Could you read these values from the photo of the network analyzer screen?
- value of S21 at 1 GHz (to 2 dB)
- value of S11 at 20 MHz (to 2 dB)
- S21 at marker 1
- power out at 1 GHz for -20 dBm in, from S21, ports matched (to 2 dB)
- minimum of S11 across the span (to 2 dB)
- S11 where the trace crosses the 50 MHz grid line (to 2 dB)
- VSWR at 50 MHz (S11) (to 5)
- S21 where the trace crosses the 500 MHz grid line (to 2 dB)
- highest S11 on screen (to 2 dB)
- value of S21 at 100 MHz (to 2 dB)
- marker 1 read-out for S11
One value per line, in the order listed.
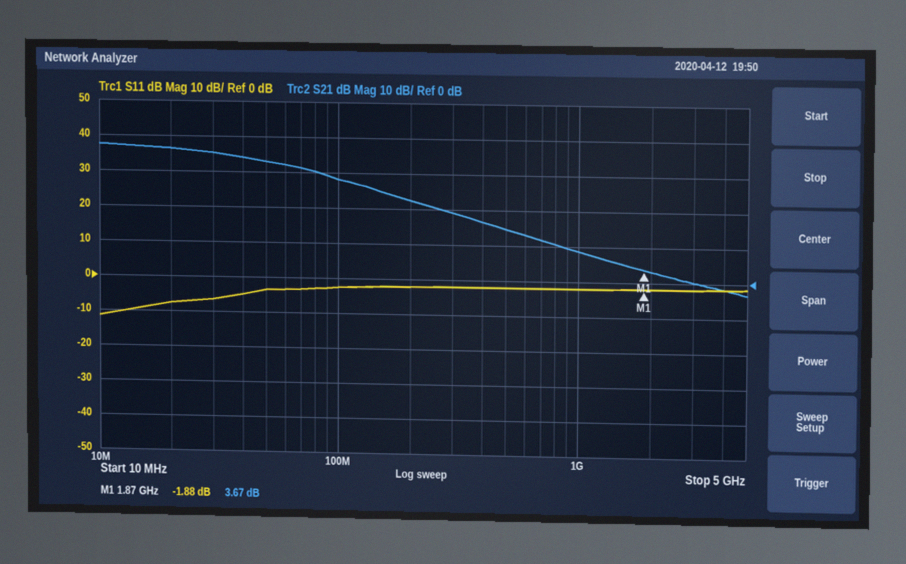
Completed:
8 dB
-8 dB
3.67 dB
-12 dBm
-12 dB
-4 dB
5
14 dB
-2 dB
28 dB
-1.88 dB
